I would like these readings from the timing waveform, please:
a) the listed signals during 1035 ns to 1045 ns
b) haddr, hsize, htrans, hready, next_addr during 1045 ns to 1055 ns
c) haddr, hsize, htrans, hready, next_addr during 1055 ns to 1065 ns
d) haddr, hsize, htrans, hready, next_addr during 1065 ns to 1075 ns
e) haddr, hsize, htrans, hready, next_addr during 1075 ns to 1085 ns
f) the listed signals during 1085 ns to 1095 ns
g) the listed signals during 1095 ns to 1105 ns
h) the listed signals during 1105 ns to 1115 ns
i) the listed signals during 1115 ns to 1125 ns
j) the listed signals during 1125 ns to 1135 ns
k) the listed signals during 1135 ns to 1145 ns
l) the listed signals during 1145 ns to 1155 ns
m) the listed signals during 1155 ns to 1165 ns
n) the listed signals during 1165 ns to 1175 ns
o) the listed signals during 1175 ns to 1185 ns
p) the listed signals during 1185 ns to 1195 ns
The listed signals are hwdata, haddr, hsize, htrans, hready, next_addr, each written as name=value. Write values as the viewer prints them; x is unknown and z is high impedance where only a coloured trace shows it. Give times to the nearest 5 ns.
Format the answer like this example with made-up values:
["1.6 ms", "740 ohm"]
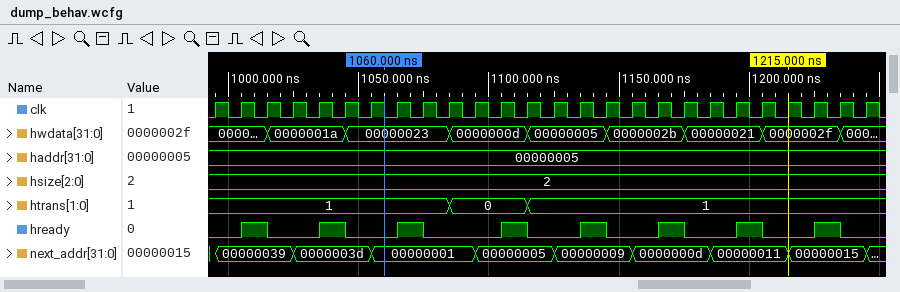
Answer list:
["hwdata=0000001a, haddr=00000005, hsize=2, htrans=1, hready=1, next_addr=0000003d", "haddr=00000005, hsize=2, htrans=1, hready=0, next_addr=0000003d", "haddr=00000005, hsize=2, htrans=1, hready=0, next_addr=00000001", "haddr=00000005, hsize=2, htrans=1, hready=1, next_addr=00000001", "haddr=00000005, hsize=2, htrans=1, hready=0, next_addr=00000001", "hwdata=0000000d, haddr=00000005, hsize=2, htrans=0, hready=0, next_addr=00000001", "hwdata=0000000d, haddr=00000005, hsize=2, htrans=0, hready=0, next_addr=00000005", "hwdata=0000000d, haddr=00000005, hsize=2, htrans=0, hready=1, next_addr=00000005", "hwdata=00000005, haddr=00000005, hsize=2, htrans=1, hready=0, next_addr=00000005", "hwdata=00000005, haddr=00000005, hsize=2, htrans=1, hready=0, next_addr=00000009", "hwdata=00000005, haddr=00000005, hsize=2, htrans=1, hready=1, next_addr=00000009", "hwdata=0000002b, haddr=00000005, hsize=2, htrans=1, hready=0, next_addr=00000009", "hwdata=0000002b, haddr=00000005, hsize=2, htrans=1, hready=0, next_addr=0000000d", "hwdata=0000002b, haddr=00000005, hsize=2, htrans=1, hready=1, next_addr=0000000d", "hwdata=00000021, haddr=00000005, hsize=2, htrans=1, hready=0, next_addr=0000000d", "hwdata=00000021, haddr=00000005, hsize=2, htrans=1, hready=0, next_addr=00000011"]
